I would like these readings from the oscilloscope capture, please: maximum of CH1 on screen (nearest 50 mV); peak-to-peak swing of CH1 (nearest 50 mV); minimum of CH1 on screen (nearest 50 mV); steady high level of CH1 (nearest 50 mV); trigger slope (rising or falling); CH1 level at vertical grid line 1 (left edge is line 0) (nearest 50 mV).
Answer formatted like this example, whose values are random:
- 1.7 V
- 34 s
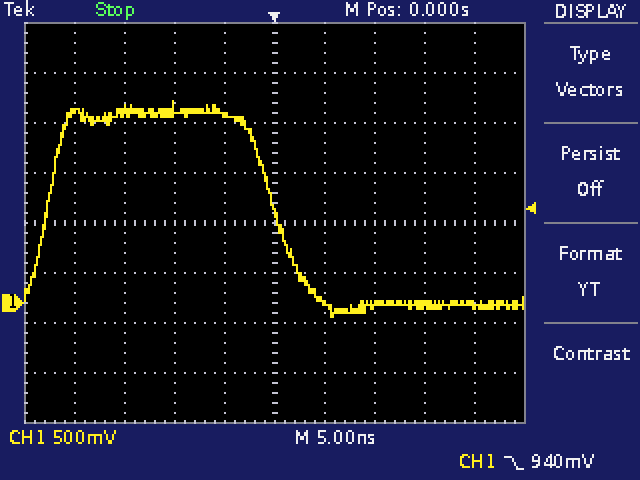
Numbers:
- 2.00 V
- 2.15 V
- -150 mV
- 1.90 V
- falling
- 1.90 V
